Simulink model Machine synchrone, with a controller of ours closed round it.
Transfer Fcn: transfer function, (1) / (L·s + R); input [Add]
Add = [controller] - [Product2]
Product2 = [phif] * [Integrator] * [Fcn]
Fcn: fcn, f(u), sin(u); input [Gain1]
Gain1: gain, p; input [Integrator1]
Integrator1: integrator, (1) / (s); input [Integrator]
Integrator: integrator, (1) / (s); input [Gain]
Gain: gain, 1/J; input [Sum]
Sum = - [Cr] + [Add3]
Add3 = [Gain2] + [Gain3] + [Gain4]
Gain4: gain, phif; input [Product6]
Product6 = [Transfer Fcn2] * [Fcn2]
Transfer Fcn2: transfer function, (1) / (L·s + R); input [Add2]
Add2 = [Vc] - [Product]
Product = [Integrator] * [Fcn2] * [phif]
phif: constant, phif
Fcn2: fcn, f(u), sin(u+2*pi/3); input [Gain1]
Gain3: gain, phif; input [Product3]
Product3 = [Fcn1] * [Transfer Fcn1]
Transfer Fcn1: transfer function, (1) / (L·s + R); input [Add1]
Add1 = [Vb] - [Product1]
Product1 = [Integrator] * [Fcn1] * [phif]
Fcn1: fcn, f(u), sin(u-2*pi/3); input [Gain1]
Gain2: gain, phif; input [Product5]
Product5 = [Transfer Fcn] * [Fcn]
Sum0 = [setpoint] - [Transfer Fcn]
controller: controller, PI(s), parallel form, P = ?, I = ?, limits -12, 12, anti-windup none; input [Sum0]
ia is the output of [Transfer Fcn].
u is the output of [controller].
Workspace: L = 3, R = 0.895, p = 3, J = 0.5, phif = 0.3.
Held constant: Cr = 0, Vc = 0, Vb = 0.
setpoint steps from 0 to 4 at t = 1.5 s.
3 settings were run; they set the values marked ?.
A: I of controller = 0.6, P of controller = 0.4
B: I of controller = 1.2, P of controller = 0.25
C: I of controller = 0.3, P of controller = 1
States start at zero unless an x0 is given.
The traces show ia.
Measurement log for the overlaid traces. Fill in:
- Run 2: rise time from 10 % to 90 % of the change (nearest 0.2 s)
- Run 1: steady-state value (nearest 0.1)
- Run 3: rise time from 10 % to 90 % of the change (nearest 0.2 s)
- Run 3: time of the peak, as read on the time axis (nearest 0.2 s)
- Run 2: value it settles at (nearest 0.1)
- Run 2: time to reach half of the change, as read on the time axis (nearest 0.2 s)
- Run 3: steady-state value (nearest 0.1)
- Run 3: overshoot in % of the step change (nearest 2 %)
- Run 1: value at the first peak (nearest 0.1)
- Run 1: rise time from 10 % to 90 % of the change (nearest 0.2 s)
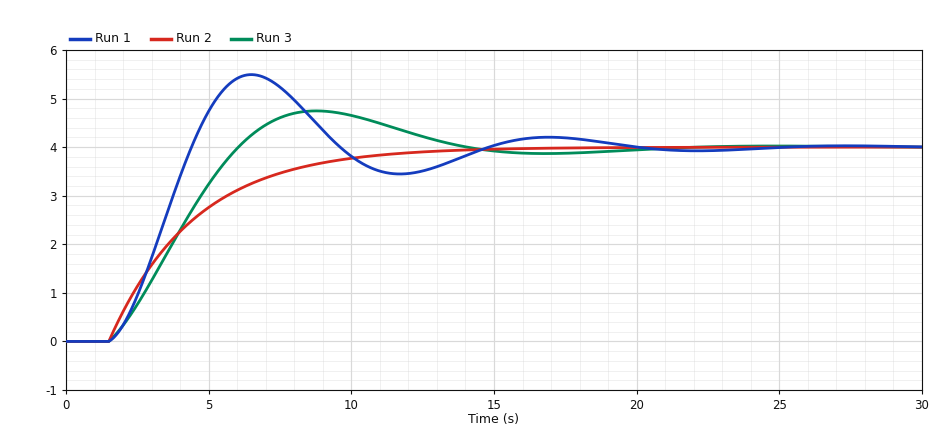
6.6 s
4.0
3.4 s
8.8 s
4.0
3.6 s
4.0
18 %
5.5
2.0 s
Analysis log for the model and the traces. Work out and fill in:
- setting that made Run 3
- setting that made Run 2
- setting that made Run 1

A
C
B
